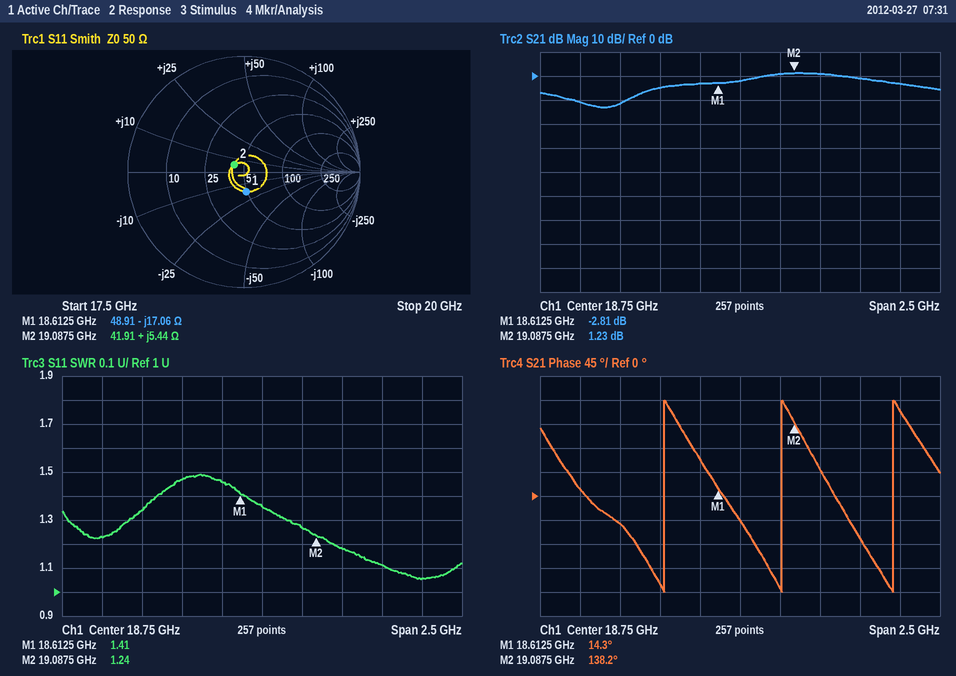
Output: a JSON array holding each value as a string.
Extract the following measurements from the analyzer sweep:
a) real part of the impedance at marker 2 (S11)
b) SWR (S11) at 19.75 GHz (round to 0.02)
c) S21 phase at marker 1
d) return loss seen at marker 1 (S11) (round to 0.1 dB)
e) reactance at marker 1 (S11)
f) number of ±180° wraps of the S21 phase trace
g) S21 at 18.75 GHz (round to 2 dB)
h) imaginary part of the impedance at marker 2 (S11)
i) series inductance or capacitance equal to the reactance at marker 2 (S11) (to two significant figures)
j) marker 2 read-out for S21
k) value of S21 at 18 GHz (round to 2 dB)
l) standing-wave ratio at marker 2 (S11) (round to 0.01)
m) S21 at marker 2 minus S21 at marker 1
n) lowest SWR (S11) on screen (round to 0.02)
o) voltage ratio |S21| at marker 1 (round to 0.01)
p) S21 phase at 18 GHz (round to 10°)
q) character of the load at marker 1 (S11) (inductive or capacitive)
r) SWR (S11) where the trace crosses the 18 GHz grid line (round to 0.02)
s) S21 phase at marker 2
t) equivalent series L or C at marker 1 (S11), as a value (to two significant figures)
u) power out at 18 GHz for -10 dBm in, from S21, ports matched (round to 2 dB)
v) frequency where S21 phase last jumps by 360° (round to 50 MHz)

["41.91 Ω", "1.06", "14.3°", "15.4 dB", "-17.06 Ω", "3", "-2 dB", "+5.44 Ω", "45 pH", "1.23 dB", "-12 dB", "1.24", "4.04 dB", "1.06", "0.72", "-50°", "capacitive", "1.34", "138.2°", "500 fF", "-22 dBm", "19.70 GHz"]
